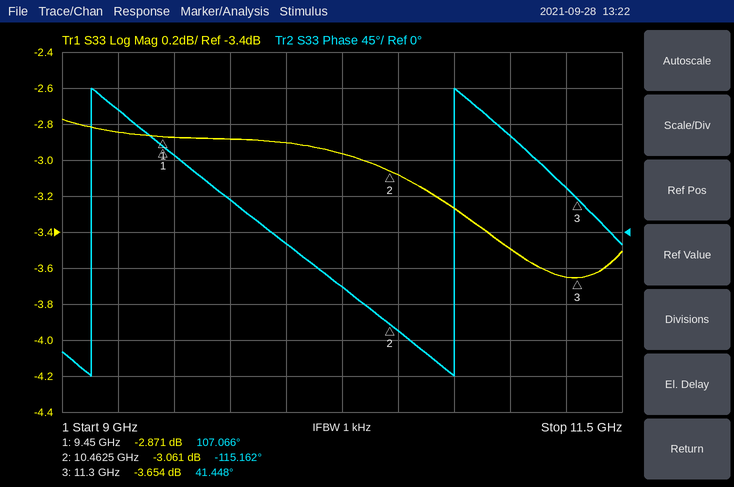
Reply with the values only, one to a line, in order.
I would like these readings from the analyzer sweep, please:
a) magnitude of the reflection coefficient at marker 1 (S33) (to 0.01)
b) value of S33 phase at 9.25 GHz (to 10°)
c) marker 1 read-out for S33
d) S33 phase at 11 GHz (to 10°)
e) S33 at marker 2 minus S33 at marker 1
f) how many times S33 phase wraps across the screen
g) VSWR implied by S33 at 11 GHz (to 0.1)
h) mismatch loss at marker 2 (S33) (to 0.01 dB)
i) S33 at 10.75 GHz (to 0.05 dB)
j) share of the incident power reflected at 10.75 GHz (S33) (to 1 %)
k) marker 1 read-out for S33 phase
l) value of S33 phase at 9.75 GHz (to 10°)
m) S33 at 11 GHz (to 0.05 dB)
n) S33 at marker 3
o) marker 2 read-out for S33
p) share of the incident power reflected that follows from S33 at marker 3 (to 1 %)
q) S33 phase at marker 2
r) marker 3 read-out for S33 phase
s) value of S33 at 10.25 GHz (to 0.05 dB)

0.72
150°
-2.871 dB
120°
-0.190 dB
2
5.0
2.96 dB
-3.25 dB
47 %
107.066°
40°
-3.50 dB
-3.654 dB
-3.061 dB
43 %
-115.162°
41.448°
-2.95 dB
